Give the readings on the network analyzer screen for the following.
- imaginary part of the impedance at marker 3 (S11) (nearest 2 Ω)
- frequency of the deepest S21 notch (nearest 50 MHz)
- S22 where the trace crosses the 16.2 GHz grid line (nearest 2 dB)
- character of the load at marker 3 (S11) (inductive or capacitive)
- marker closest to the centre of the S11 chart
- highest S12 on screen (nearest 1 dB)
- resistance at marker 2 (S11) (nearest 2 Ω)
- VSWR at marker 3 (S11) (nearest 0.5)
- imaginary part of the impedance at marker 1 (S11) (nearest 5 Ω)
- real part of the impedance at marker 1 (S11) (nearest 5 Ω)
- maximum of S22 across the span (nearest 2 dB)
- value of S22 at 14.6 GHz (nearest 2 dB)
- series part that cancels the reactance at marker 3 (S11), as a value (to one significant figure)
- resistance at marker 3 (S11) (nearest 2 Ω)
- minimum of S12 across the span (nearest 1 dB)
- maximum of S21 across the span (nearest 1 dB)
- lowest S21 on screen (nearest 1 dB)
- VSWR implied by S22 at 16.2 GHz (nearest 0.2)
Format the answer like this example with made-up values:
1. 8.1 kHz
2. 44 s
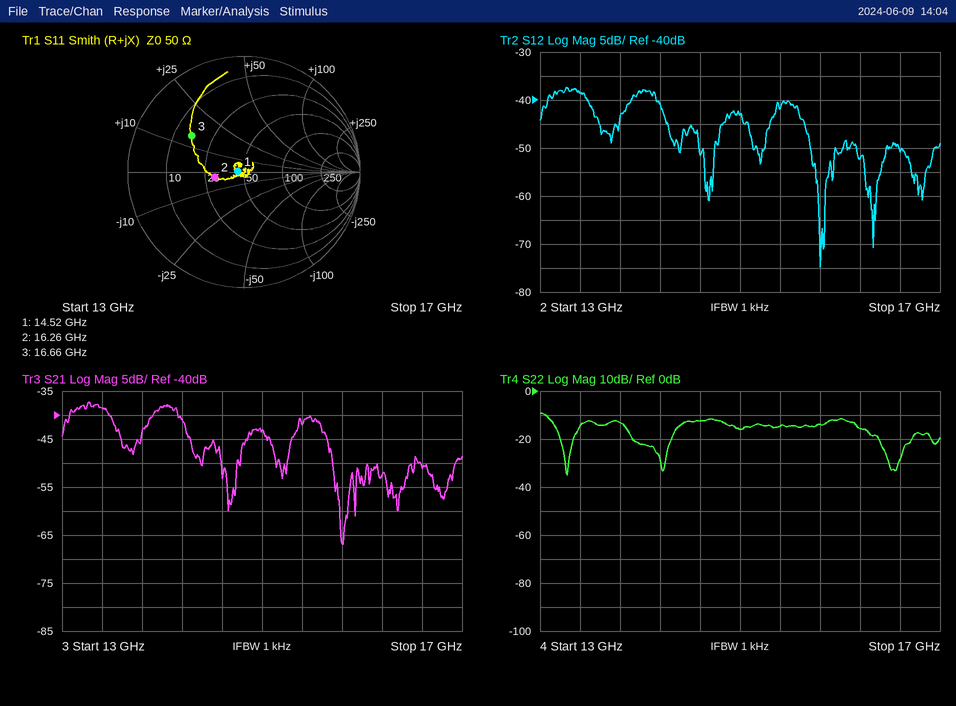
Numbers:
1. +14 Ω
2. 15.80 GHz
3. -16 dB
4. inductive
5. marker 1
6. -37 dB
7. 30 Ω
8. 3.5
9. 0 Ω
10. 45 Ω
11. -10 dB
12. -12 dB
13. 700 fF
14. 16 Ω
15. -75 dB
16. -37 dB
17. -67 dB
18. 1.4
